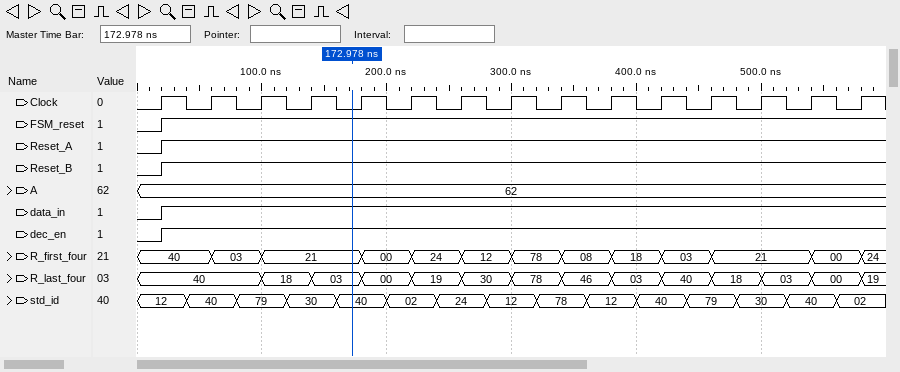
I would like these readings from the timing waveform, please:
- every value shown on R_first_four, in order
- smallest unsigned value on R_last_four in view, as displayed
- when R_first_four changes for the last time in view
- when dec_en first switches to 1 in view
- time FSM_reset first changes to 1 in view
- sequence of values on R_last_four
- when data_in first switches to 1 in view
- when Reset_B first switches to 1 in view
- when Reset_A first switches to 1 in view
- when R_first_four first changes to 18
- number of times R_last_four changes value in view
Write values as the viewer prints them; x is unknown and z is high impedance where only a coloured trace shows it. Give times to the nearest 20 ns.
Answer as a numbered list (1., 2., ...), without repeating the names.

1. 40, 03, 21, 00, 24, 12, 78, 08, 18, 03, 21, 00, 24
2. 00
3. 580 ns
4. 20 ns
5. 20 ns
6. 40, 18, 03, 00, 19, 30, 78, 46, 03, 40, 18, 03, 00, 19
7. 20 ns
8. 20 ns
9. 20 ns
10. 380 ns
11. 13
